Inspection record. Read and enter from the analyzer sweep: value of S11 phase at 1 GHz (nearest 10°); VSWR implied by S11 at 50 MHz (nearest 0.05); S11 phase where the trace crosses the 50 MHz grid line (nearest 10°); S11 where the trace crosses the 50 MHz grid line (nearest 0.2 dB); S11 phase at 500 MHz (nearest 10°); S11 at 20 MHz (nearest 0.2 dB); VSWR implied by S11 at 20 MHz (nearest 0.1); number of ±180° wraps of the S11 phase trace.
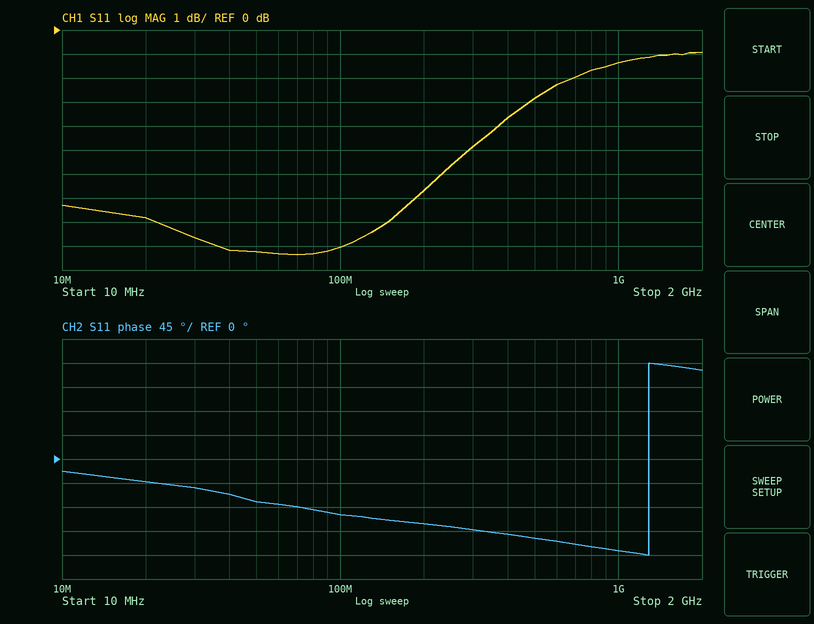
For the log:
-170°
2.05
-80°
-9.2 dB
-150°
-7.8 dB
2.4
1
